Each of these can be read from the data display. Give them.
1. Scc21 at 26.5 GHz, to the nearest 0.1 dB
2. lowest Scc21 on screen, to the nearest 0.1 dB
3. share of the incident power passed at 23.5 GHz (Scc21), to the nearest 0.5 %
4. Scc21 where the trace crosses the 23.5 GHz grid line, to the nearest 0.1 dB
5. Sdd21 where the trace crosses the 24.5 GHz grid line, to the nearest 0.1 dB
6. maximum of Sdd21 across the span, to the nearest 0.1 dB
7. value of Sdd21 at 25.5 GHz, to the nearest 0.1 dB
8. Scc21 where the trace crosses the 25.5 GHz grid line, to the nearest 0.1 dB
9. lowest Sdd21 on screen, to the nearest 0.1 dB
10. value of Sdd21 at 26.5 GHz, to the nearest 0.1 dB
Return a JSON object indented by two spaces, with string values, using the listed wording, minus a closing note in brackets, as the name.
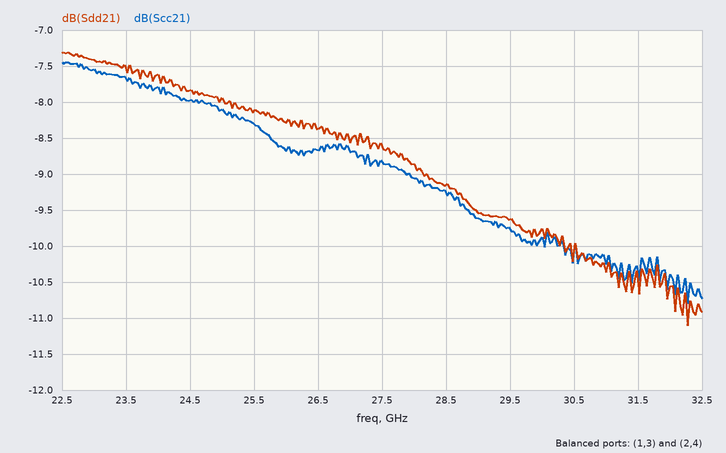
{
  "Scc21 at 26.5 GHz, to the nearest 0.1 dB": "-8.7 dB",
  "lowest Scc21 on screen, to the nearest 0.1 dB": "-10.8 dB",
  "share of the incident power passed at 23.5 GHz (Scc21), to the nearest 0.5 %": "17.0 %",
  "Scc21 where the trace crosses the 23.5 GHz grid line, to the nearest 0.1 dB": "-7.7 dB",
  "Sdd21 where the trace crosses the 24.5 GHz grid line, to the nearest 0.1 dB": "-7.8 dB",
  "maximum of Sdd21 across the span, to the nearest 0.1 dB": "-7.3 dB",
  "value of Sdd21 at 25.5 GHz, to the nearest 0.1 dB": "-8.1 dB",
  "Scc21 where the trace crosses the 25.5 GHz grid line, to the nearest 0.1 dB": "-8.3 dB",
  "lowest Sdd21 on screen, to the nearest 0.1 dB": "-11.1 dB",
  "value of Sdd21 at 26.5 GHz, to the nearest 0.1 dB": "-8.4 dB"
}
